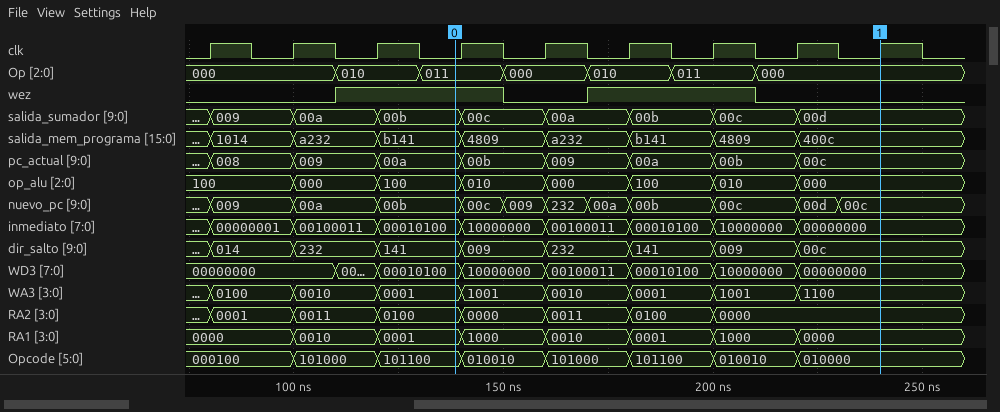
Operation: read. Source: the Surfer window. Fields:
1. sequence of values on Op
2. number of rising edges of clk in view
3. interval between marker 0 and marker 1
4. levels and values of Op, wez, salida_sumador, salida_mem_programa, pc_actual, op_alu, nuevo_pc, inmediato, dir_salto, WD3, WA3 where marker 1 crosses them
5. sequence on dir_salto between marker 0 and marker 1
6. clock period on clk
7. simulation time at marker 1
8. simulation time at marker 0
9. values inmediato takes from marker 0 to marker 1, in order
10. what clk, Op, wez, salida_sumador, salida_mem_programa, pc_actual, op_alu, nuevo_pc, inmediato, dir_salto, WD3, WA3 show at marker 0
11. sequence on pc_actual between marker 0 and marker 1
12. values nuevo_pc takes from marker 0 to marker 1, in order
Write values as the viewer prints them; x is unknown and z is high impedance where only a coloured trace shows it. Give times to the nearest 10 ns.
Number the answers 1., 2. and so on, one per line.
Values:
1. 000, 010, 011, 000, 010, 011, 000
2. 9
3. 100 ns
4. Op=000, wez=0, salida_sumador=00d, salida_mem_programa=400c, pc_actual=00c, op_alu=000, nuevo_pc=00c, inmediato=00000000, dir_salto=00c, WD3=00000000, WA3=1100
5. 141, 009, 232, 141, 009, 00c
6. 20 ns
7. 240 ns
8. 140 ns
9. 00010100, 10000000, 00100011, 00010100, 10000000, 00000000
10. clk=0, Op=011, wez=1, salida_sumador=00b, salida_mem_programa=b141, pc_actual=00a, op_alu=100, nuevo_pc=00b, inmediato=00010100, dir_salto=141, WD3=00010100, WA3=0001
11. 00a, 00b, 009, 00a, 00b, 00c
12. 00b, 00c, 009, 232, 00a, 00b, 00c, 00d, 00c
